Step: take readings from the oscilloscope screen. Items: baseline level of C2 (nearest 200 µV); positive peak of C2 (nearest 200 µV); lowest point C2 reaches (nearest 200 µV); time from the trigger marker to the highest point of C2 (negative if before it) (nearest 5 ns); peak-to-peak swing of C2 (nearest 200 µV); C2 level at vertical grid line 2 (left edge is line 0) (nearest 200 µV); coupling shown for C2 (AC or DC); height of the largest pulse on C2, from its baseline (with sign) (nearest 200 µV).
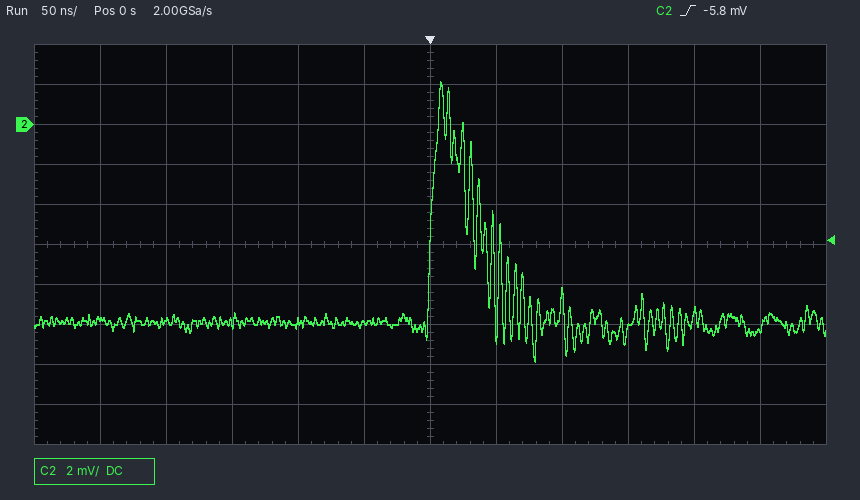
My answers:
-9.8 mV
2.2 mV
-11.8 mV
+10 ns
14.0 mV
-9.8 mV
DC
+12.0 mV
